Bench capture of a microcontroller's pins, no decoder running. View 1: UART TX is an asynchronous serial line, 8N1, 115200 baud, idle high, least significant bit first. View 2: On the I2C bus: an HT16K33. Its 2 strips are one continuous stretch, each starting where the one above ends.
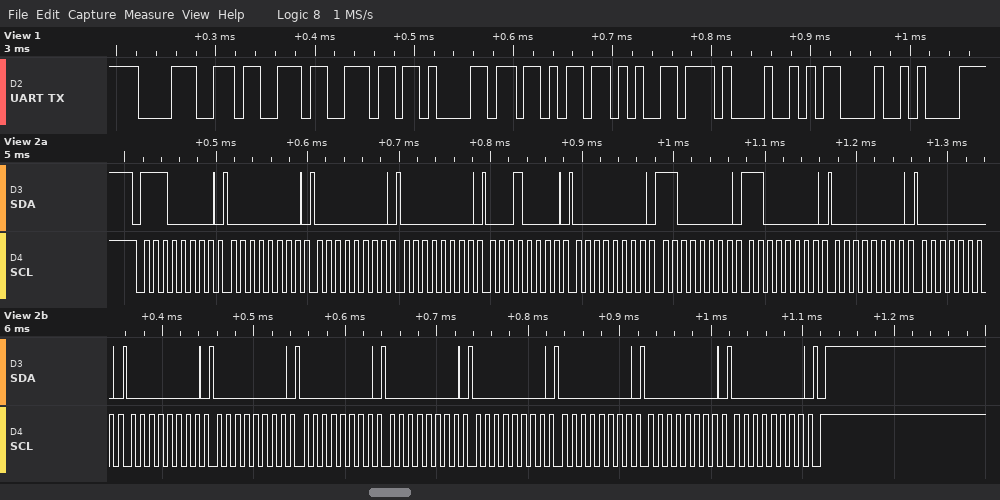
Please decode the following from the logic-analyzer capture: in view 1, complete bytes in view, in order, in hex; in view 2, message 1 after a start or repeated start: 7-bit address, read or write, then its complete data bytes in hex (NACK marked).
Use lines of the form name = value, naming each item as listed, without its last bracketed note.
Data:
in view 1, complete bytes in view, in order, in hex = 0x38 0x73 0x6E 0x61 0x6B 0x65 0x21 0x0D 0x0A
in view 2, message 1 after a start or repeated start: 7-bit address, read or write, then its complete data bytes in hex = 0x70 write: 00 00 00 10 00 C0 C0 00 00 00 00 00 00 00 00 00 00
